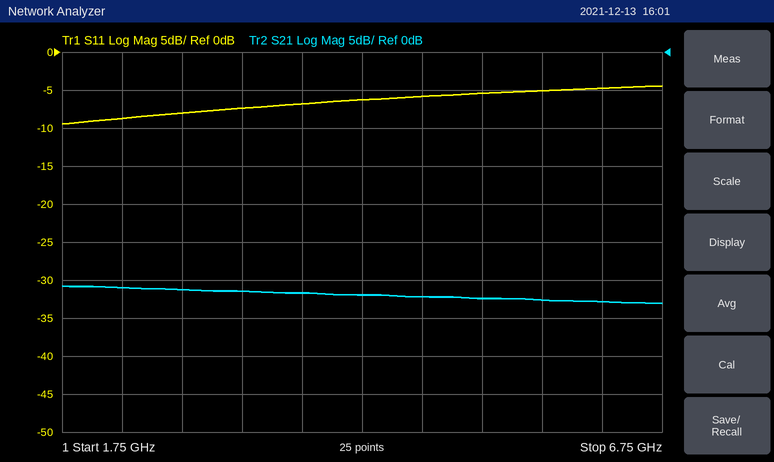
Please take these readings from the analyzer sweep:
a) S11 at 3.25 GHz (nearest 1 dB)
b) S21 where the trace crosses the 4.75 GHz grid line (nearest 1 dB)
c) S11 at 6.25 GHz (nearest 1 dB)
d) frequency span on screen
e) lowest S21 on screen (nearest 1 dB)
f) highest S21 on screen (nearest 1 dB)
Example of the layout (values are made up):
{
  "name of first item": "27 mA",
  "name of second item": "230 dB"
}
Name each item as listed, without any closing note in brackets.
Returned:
{
  "S11 at 3.25 GHz": "-7 dB",
  "S21 where the trace crosses the 4.75 GHz grid line": "-32 dB",
  "S11 at 6.25 GHz": "-5 dB",
  "frequency span on screen": "5 GHz",
  "lowest S21 on screen": "-33 dB",
  "highest S21 on screen": "-31 dB"
}
